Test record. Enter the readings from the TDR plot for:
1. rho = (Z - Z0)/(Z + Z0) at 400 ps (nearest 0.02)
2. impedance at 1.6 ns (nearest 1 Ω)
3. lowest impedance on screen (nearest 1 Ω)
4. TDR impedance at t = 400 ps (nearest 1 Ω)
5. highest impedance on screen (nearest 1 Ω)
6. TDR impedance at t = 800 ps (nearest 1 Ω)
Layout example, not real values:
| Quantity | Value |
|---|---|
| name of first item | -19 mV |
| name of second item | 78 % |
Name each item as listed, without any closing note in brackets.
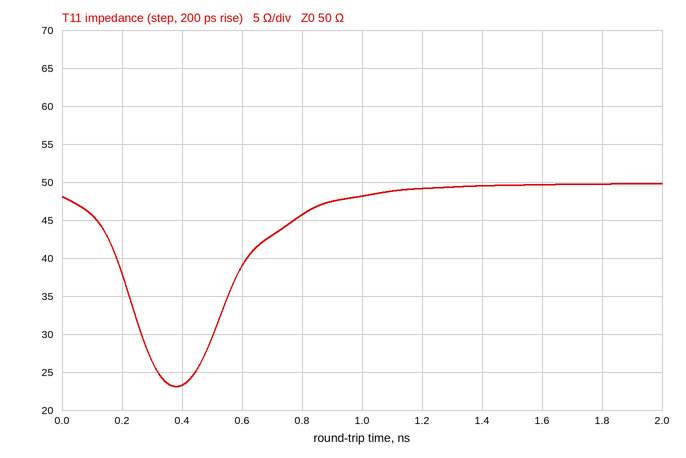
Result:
| Quantity | Value |
|---|---|
| rho = (Z - Z0)/(Z + Z0) at 400 ps | -0.36 |
| impedance at 1.6 ns | 50 Ω |
| lowest impedance on screen | 23 Ω |
| TDR impedance at t = 400 ps | 23 Ω |
| highest impedance on screen | 50 Ω |
| TDR impedance at t = 800 ps | 46 Ω |
